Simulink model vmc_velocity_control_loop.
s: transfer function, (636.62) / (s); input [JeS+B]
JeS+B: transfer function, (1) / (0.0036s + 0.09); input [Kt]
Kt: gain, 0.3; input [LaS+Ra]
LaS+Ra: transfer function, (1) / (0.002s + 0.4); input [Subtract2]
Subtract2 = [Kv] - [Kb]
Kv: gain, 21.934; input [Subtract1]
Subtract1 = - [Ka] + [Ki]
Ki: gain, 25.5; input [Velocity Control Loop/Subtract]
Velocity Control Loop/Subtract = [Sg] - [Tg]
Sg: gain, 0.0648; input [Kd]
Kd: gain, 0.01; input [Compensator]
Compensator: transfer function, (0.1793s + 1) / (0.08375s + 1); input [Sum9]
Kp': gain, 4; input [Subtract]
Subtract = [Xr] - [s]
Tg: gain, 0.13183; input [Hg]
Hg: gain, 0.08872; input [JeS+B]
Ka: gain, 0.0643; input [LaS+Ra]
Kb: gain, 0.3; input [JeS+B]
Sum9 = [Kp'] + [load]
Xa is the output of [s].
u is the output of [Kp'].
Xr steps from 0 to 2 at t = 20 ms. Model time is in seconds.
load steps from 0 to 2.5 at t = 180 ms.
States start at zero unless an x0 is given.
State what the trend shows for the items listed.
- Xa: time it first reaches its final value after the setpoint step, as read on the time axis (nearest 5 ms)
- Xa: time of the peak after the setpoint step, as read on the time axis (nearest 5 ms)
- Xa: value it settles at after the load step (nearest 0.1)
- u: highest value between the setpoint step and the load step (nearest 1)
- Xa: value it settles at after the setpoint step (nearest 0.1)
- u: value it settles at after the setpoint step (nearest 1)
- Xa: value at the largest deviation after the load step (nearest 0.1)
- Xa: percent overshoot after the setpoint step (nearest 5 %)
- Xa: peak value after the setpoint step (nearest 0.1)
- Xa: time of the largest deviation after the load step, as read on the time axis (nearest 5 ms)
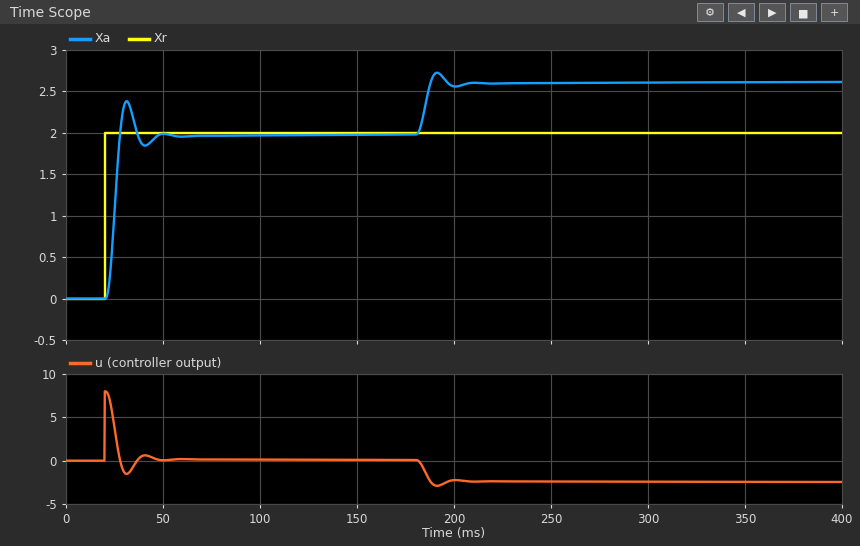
30 ms
30 ms
2.6
8
2.0
0
2.7
20 %
2.4
190 ms
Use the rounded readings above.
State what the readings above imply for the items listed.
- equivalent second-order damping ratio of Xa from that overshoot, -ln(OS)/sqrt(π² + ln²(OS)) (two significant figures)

0.46
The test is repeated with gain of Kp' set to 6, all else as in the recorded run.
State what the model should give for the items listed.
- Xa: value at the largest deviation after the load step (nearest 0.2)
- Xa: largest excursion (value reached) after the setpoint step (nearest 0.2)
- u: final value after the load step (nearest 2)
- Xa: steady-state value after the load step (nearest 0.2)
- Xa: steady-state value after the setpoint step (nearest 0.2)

2.6
2.8
-2
2.4
2.0
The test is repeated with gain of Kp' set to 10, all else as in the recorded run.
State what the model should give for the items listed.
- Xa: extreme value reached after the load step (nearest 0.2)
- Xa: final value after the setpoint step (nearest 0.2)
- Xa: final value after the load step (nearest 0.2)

2.4
2.0
2.2
